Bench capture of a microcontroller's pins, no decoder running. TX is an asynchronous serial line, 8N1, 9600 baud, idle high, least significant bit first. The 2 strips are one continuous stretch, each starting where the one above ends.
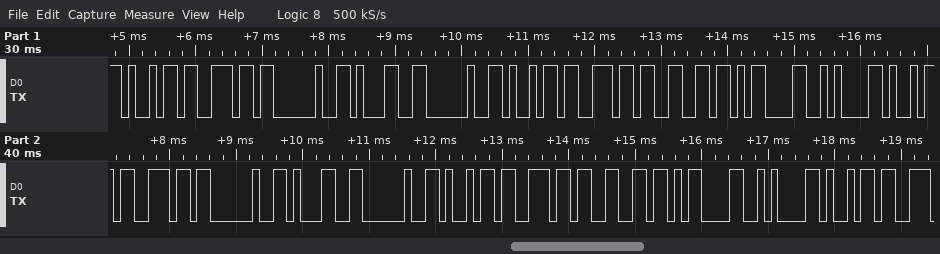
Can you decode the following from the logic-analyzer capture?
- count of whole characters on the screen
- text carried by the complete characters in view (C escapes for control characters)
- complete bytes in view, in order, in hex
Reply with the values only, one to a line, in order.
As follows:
21
"in 1 inf\r\nin 1 inf\r\ni"
69 6E 20 31 20 69 6E 66 0D 0A 69 6E 20 31 20 69 6E 66 0D 0A 69
